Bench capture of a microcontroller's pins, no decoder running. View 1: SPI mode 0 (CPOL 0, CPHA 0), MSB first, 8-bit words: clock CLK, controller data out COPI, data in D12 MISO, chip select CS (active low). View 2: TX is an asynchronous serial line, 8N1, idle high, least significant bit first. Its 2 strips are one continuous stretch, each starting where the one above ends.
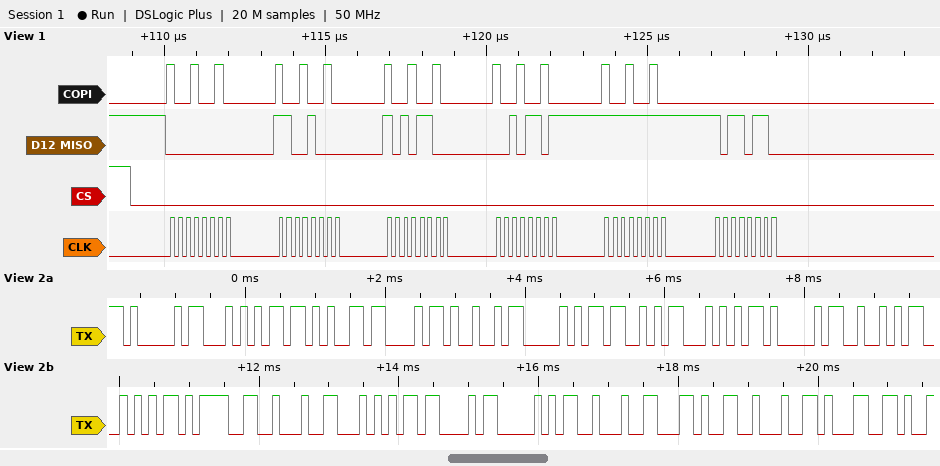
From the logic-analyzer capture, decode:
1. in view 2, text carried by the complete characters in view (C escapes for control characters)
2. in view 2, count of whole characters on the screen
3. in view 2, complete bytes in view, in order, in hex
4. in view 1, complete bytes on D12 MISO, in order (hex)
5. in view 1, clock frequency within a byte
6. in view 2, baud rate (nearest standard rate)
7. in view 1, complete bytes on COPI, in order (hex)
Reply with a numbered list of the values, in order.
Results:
1. "AT+CIPSTART=\"TCP\",\"1"
2. 20
3. 41 54 2B 43 49 50 53 54 41 52 54 3D 22 54 43 50 22 2C 22 31
4. 00 C8 AC 2D FF B6
5. 4 MHz
6. 9600 baud
7. 92 92 92 92 92 00
